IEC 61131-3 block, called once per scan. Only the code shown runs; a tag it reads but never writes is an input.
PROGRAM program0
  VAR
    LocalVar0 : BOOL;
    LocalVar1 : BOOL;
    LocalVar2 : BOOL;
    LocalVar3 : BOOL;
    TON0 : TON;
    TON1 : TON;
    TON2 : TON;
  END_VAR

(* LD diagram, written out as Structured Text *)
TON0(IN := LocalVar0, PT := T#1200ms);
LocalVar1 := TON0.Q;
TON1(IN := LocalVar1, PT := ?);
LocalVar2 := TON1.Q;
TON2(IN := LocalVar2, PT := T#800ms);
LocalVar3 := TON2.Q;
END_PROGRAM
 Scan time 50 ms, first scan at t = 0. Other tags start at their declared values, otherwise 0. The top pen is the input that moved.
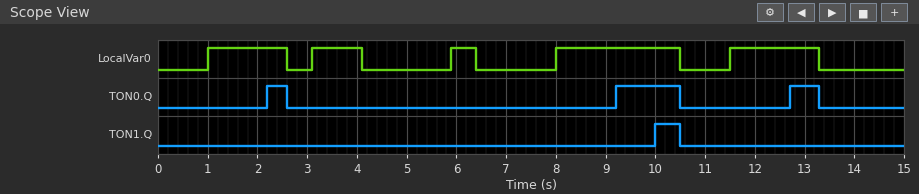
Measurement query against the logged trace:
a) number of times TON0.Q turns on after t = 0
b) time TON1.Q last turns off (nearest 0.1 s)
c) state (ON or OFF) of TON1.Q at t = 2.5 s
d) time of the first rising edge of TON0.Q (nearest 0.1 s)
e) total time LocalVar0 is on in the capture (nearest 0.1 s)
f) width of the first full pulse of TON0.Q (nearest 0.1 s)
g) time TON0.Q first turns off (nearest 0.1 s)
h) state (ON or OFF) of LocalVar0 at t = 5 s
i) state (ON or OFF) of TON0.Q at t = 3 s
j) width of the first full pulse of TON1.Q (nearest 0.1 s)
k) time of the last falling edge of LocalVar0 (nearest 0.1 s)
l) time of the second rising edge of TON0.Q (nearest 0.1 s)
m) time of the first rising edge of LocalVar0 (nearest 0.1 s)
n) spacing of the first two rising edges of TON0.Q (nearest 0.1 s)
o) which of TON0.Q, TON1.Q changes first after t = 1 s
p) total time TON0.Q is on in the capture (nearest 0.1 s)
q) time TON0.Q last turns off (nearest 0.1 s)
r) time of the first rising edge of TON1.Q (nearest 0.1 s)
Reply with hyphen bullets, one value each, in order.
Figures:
- 3
- 10.5 s
- OFF
- 2.2 s
- 7.4 s
- 0.4 s
- 2.6 s
- OFF
- OFF
- 0.5 s
- 13.3 s
- 9.2 s
- 1.0 s
- 7.0 s
- TON0.Q
- 2.3 s
- 13.3 s
- 10.0 s
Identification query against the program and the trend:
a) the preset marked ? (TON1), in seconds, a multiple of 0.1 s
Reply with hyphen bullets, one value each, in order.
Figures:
- 0.8 s
